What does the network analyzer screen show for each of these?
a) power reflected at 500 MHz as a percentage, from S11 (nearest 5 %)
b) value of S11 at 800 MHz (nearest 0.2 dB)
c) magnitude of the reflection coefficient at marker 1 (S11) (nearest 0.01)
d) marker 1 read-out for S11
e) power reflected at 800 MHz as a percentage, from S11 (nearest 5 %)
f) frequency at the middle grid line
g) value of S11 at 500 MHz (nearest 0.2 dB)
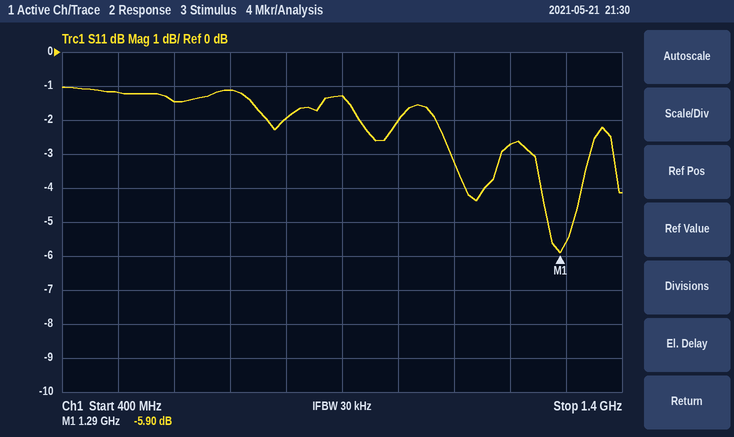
75 %
-2.0 dB
0.51
-5.90 dB
65 %
900 MHz
-1.2 dB
